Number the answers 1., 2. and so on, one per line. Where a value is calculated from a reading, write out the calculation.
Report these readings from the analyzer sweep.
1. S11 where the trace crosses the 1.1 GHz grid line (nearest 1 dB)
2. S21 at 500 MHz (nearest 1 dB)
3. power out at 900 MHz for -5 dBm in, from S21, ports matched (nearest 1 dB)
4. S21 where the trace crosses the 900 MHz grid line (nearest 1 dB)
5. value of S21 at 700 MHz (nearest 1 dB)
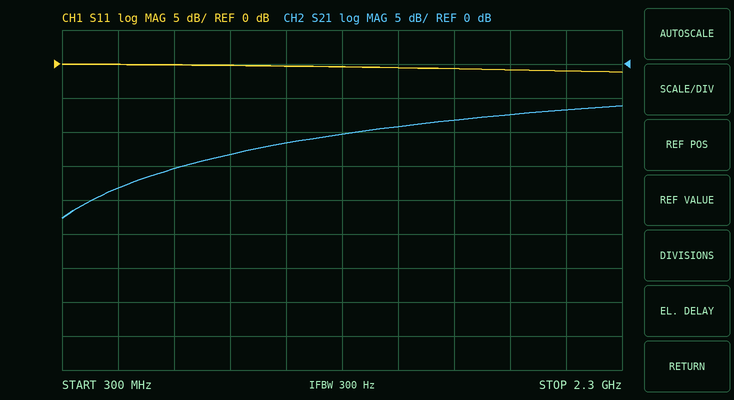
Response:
1. 0 dB
2. -18 dB
3. -5 dBm + (-13 dB) = -18 dBm
4. -13 dB
5. -15 dB
